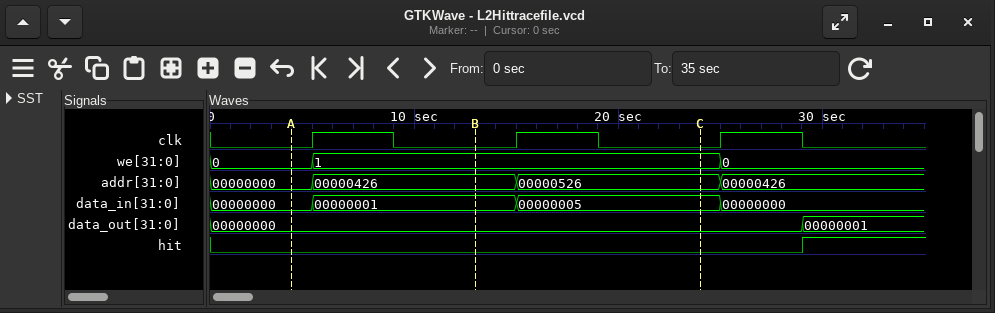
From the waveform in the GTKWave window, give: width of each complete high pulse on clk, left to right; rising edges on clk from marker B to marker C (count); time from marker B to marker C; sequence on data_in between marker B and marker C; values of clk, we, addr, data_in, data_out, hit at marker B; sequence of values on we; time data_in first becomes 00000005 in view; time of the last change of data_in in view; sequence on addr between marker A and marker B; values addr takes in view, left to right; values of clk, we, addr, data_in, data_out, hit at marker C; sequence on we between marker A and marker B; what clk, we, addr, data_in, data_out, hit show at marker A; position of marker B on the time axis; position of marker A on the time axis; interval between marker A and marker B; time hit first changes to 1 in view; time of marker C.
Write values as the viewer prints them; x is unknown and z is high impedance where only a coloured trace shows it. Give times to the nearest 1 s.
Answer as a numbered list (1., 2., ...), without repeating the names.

1. 4 s, 4 s, 4 s
2. 1
3. 11 s
4. 00000001, 00000005
5. clk=0, we=1, addr=00000426, data_in=00000001, data_out=00000000, hit=0
6. 0, 1, 0
7. 15 s
8. 25 s
9. 00000000, 00000426
10. 00000000, 00000426, 00000526, 00000426
11. clk=0, we=1, addr=00000526, data_in=00000005, data_out=00000000, hit=0
12. 0, 1
13. clk=0, we=0, addr=00000000, data_in=00000000, data_out=00000000, hit=0
14. 13 s
15. 4 s
16. 9 s
17. 29 s
18. 24 s
